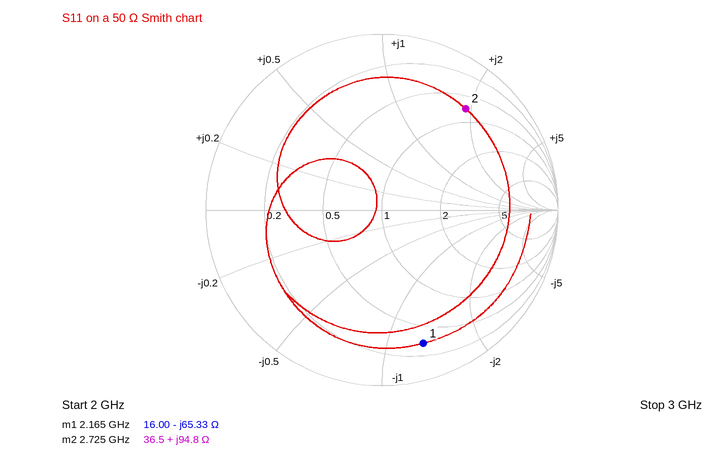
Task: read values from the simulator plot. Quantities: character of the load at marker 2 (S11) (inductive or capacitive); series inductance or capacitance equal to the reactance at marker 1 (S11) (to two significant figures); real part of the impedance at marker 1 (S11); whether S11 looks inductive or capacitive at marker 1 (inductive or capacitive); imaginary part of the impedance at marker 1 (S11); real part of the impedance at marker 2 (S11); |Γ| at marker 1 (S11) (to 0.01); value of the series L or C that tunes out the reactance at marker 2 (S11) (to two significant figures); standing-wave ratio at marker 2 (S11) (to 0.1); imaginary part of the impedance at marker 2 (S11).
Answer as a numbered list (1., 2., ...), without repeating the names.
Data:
1. inductive
2. 1.1 pF
3. 16.00 Ω
4. capacitive
5. -65.33 Ω
6. 36.5 Ω
7. 0.79
8. 620 fF
9. 6.9
10. +94.8 Ω
